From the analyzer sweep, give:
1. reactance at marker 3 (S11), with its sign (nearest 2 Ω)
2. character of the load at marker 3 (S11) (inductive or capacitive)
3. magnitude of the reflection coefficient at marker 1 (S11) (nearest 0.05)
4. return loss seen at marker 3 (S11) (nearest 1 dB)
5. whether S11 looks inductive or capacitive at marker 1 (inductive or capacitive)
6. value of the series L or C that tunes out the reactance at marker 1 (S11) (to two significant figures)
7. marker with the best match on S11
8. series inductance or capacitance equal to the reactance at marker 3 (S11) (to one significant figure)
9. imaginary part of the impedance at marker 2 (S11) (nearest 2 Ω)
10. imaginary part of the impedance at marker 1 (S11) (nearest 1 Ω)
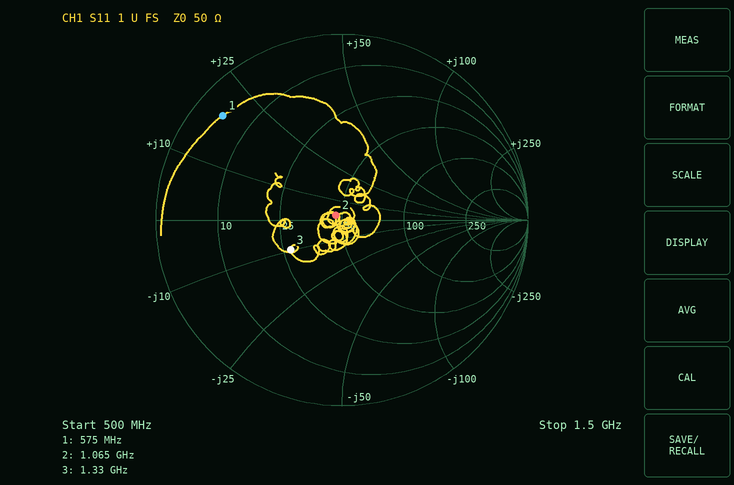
-10 Ω
capacitive
0.85
10 dB
inductive
15 pF
marker 2
10 pF
+2 Ω
+19 Ω
